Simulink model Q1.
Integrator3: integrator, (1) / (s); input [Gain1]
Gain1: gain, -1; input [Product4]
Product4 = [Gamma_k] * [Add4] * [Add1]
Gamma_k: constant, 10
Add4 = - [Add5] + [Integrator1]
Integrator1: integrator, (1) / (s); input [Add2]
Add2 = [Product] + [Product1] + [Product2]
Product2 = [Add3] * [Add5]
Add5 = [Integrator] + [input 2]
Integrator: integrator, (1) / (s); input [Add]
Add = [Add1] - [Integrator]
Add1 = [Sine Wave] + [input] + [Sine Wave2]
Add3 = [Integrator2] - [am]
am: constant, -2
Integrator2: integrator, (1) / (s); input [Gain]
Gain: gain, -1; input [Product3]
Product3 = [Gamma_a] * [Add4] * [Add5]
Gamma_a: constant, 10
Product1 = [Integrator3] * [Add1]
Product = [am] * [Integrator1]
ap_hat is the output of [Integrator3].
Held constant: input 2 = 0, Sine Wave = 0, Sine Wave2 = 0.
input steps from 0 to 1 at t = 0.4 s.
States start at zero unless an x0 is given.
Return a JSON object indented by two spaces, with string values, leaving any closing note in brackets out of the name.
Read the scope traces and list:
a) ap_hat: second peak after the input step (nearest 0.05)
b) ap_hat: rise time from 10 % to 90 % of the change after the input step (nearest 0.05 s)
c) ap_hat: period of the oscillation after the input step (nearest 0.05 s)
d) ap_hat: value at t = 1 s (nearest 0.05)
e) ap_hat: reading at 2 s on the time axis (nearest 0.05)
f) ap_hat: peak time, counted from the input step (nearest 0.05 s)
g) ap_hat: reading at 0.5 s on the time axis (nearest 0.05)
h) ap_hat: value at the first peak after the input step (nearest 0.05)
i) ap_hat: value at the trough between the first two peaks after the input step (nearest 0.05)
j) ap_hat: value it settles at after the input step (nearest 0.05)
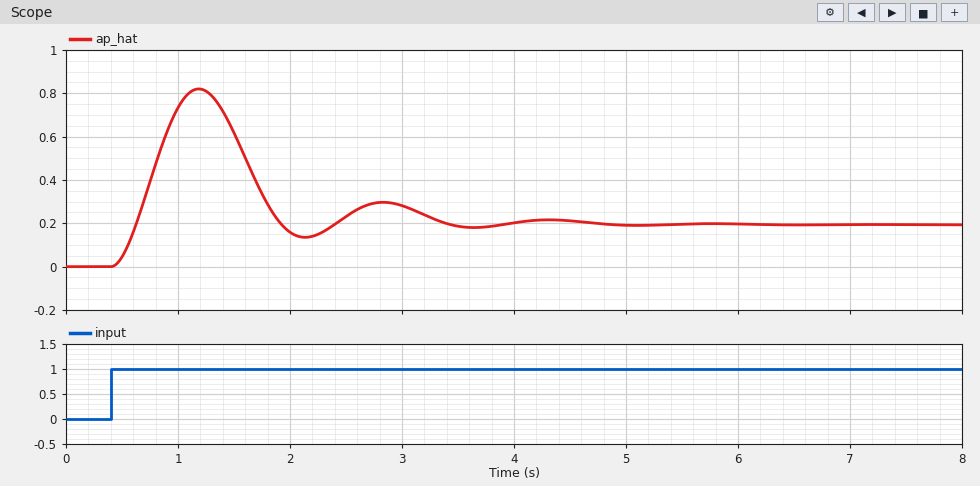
{
  "ap_hat: second peak after the input step": "0.30",
  "ap_hat: rise time from 10 % to 90 % of the change after the input step": "0.15 s",
  "ap_hat: period of the oscillation after the input step": "1.65 s",
  "ap_hat: value at t = 1 s": "0.75",
  "ap_hat: reading at 2 s on the time axis": "0.15",
  "ap_hat: peak time, counted from the input step": "0.80 s",
  "ap_hat: reading at 0.5 s on the time axis": "0.05",
  "ap_hat: value at the first peak after the input step": "0.80",
  "ap_hat: value at the trough between the first two peaks after the input step": "0.15",
  "ap_hat: value it settles at after the input step": "0.20"
}
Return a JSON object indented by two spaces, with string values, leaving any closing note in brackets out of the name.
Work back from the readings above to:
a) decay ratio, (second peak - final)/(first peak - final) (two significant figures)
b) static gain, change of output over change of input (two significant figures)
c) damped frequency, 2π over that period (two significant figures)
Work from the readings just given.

{
  "decay ratio, (second peak - final)/(first peak - final)": "0.17",
  "static gain, change of output over change of input": "0.20",
  "damped frequency, 2π over that period": "3.8 rad/s"
}
